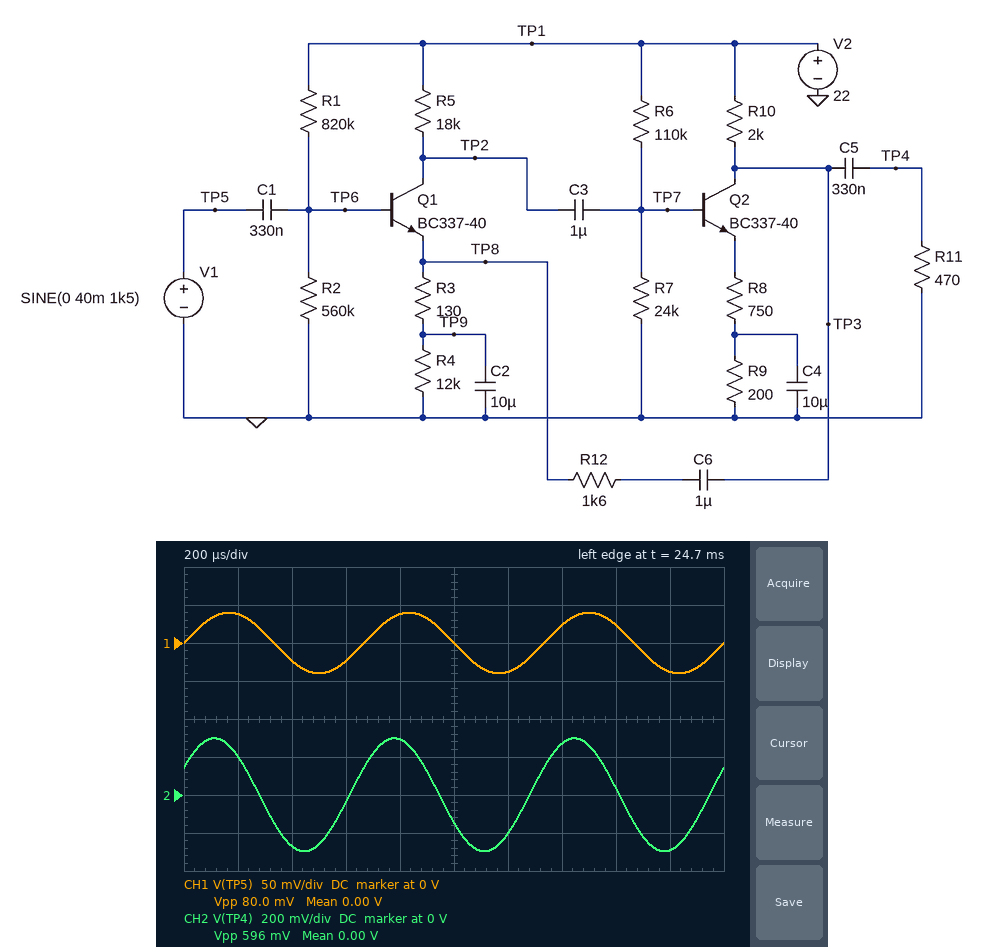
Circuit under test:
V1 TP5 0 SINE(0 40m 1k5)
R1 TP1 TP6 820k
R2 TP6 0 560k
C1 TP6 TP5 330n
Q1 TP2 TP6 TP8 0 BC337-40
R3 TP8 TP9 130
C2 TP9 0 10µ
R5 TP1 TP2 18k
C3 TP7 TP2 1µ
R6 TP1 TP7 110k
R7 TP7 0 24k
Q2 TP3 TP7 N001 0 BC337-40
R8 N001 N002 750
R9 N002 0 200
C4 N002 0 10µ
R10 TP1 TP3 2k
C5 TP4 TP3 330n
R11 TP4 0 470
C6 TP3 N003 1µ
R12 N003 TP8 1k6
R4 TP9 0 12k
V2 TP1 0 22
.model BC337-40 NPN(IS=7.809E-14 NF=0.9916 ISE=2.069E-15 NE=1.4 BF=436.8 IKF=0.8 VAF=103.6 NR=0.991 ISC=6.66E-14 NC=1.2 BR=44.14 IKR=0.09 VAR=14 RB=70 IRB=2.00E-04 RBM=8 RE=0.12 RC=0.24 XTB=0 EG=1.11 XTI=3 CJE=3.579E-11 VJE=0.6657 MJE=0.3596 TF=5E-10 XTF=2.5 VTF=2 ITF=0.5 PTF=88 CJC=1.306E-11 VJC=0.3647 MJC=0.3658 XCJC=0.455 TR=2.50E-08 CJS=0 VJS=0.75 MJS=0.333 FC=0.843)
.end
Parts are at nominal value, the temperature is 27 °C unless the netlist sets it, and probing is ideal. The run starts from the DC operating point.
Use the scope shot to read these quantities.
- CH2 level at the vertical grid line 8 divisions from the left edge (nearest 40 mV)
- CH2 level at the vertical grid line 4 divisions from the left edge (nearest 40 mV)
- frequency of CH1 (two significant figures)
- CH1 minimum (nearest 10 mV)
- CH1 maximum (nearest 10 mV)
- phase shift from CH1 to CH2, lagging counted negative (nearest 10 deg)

40 mV
280 mV
1.5 kHz
-40 mV
40 mV
30 deg
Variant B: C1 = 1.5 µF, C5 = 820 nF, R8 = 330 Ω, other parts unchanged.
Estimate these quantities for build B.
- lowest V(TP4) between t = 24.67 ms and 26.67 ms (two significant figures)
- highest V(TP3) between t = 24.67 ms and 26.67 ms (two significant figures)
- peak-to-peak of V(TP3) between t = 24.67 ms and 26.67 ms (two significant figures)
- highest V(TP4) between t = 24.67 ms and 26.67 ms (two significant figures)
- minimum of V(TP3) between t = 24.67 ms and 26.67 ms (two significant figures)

-410 mV
11 V
850 mV
410 mV
10 V
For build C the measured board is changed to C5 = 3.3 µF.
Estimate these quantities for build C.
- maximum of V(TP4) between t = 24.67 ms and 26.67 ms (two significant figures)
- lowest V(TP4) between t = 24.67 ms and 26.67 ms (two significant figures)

340 mV
-340 mV
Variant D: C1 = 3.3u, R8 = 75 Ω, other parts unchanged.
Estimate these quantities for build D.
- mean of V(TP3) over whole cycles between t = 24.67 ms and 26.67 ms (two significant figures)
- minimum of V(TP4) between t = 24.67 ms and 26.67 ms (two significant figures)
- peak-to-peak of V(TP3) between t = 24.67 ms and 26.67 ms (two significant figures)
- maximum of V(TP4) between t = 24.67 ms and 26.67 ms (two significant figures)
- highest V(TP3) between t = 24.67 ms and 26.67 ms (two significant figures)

3.2 V
-400 mV
920 mV
400 mV
3.7 V
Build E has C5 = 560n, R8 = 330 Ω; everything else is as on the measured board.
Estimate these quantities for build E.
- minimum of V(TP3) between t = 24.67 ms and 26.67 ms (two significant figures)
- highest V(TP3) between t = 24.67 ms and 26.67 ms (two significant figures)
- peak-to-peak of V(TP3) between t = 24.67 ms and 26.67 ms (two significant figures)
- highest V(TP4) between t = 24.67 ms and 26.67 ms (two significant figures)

10 V
11 V
850 mV
400 mV
